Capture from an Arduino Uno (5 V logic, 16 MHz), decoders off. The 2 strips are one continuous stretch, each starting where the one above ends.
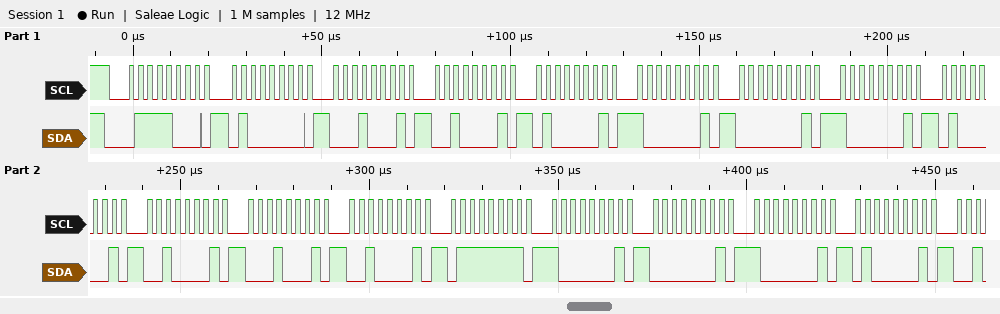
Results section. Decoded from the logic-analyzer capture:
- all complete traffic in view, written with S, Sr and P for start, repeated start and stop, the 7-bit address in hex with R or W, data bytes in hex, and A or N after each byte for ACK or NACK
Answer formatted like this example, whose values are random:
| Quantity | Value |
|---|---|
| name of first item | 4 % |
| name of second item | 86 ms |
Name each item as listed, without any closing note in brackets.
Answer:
| Quantity | Value |
|---|---|
| all complete traffic in view, written with S, Sr and P for start, repeated start and stop, the 7-bit address in hex with R or W, data bytes in hex, and A or N after each byte for ACK or NACK | S 3CW A 40 A 11 A 21 A 41 A 81 A 01 A 81 A 41 A 21 A 11 A 21 A 7F A 81 A 01 A 81 A 41 A |
